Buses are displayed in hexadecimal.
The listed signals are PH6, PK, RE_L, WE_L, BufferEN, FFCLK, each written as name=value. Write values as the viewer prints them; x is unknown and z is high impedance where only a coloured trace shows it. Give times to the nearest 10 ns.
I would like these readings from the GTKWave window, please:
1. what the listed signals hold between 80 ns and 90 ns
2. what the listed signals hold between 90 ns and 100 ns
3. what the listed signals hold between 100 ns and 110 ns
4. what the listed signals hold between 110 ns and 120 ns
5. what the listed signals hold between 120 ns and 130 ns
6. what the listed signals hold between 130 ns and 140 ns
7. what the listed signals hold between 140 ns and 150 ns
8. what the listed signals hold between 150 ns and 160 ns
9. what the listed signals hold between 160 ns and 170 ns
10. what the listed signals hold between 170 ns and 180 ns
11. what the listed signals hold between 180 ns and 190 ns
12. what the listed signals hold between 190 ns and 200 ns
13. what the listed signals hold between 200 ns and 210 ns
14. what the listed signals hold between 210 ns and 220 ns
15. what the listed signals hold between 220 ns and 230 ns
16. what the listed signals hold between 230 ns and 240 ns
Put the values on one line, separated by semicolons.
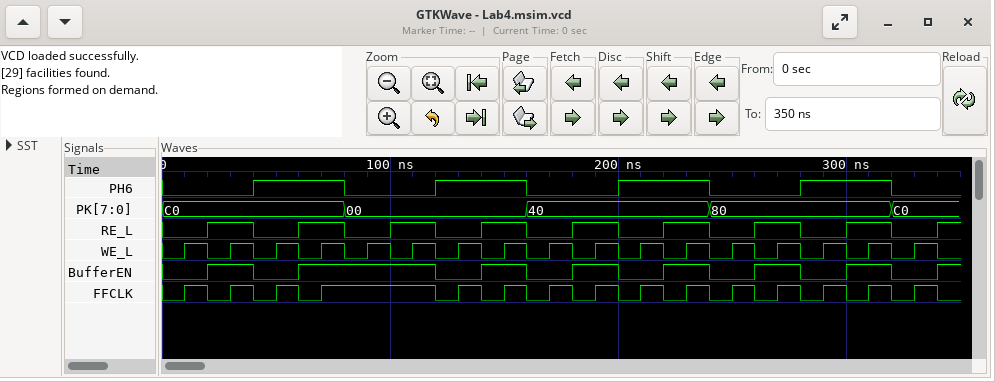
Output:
PH6=0, PK=00, RE_L=0, WE_L=0, BufferEN=1, FFCLK=1; PH6=0, PK=00, RE_L=0, WE_L=1, BufferEN=1, FFCLK=1; PH6=0, PK=00, RE_L=1, WE_L=0, BufferEN=1, FFCLK=1; PH6=0, PK=00, RE_L=1, WE_L=1, BufferEN=1, FFCLK=1; PH6=1, PK=00, RE_L=0, WE_L=0, BufferEN=0, FFCLK=0; PH6=1, PK=00, RE_L=0, WE_L=1, BufferEN=0, FFCLK=1; PH6=1, PK=00, RE_L=1, WE_L=0, BufferEN=1, FFCLK=0; PH6=1, PK=00, RE_L=1, WE_L=1, BufferEN=1, FFCLK=1; PH6=0, PK=40, RE_L=0, WE_L=0, BufferEN=0, FFCLK=0; PH6=0, PK=40, RE_L=0, WE_L=1, BufferEN=0, FFCLK=1; PH6=0, PK=40, RE_L=1, WE_L=0, BufferEN=1, FFCLK=0; PH6=0, PK=40, RE_L=1, WE_L=1, BufferEN=1, FFCLK=1; PH6=1, PK=40, RE_L=0, WE_L=0, BufferEN=0, FFCLK=0; PH6=1, PK=40, RE_L=0, WE_L=1, BufferEN=0, FFCLK=1; PH6=1, PK=40, RE_L=1, WE_L=0, BufferEN=1, FFCLK=0; PH6=1, PK=40, RE_L=1, WE_L=1, BufferEN=1, FFCLK=1
